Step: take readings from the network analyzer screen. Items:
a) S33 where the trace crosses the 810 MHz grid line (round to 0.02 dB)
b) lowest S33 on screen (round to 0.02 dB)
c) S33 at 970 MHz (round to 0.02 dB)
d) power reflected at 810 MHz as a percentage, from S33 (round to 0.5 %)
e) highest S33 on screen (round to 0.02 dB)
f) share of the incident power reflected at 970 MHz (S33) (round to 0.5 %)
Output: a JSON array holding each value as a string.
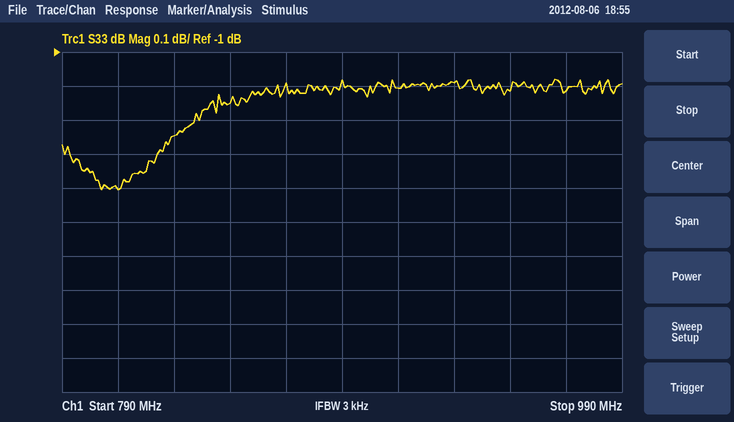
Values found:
["-1.40 dB", "-1.40 dB", "-1.12 dB", "72.5 %", "-1.08 dB", "77.5 %"]
